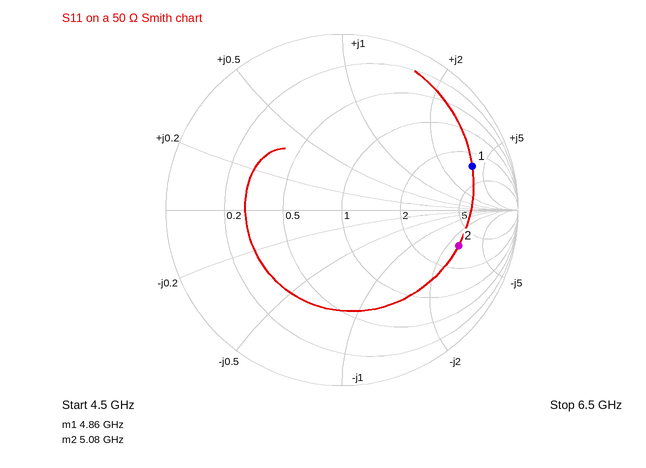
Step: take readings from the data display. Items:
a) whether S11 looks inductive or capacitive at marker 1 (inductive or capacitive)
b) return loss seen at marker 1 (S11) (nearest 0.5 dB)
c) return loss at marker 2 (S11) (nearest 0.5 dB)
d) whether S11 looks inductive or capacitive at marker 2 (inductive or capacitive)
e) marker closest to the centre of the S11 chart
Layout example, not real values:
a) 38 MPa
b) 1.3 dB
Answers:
a) inductive
b) 2.0 dB
c) 3.0 dB
d) capacitive
e) marker 2
